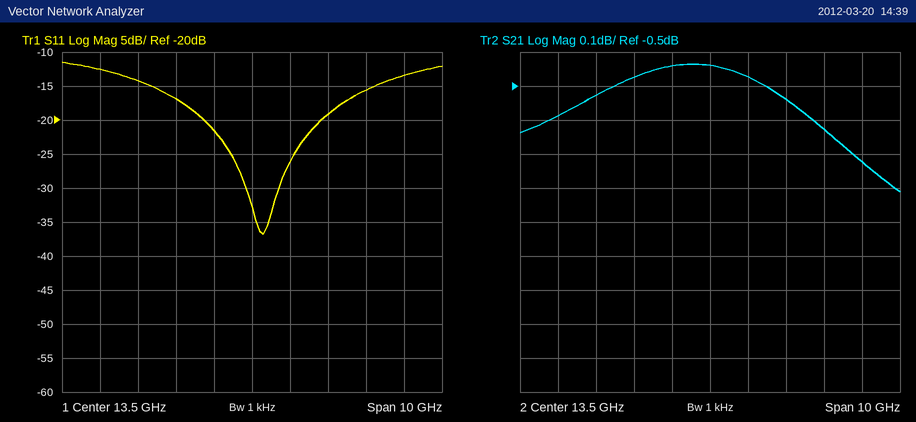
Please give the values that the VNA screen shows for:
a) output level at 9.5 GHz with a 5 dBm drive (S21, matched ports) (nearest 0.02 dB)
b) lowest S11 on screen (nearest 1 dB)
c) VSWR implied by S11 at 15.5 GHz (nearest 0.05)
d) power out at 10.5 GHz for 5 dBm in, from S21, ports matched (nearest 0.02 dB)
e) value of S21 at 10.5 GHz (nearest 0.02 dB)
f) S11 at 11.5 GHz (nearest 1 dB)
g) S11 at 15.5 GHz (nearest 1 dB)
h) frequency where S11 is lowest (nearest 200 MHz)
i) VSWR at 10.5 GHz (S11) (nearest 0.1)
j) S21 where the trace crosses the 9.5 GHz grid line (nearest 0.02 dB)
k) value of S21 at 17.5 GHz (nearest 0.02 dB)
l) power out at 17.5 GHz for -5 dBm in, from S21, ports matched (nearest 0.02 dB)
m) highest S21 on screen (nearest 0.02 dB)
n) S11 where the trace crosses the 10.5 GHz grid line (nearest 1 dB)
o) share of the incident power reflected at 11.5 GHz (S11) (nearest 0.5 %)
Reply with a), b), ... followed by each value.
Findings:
a) 4.42 dBm
b) -37 dB
c) 1.25
d) 4.48 dBm
e) -0.52 dB
f) -17 dB
g) -19 dB
h) 13.8 GHz
i) 1.5
j) -0.58 dB
k) -0.72 dB
l) -5.72 dBm
m) -0.44 dB
n) -14 dB
o) 2.0 %
